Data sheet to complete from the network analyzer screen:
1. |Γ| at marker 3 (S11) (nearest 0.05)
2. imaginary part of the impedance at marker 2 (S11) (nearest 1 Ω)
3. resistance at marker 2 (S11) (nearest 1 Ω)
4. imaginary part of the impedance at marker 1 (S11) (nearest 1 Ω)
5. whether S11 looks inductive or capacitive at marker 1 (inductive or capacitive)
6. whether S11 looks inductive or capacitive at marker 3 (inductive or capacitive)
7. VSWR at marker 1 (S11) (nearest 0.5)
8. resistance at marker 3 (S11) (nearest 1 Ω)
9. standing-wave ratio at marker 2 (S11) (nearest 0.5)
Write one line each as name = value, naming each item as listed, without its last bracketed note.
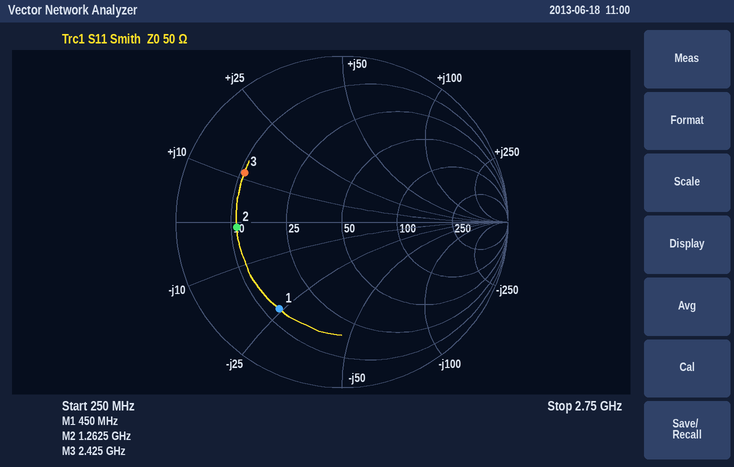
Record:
|Γ| at marker 3 (S11) = 0.65
imaginary part of the impedance at marker 2 (S11) = -1 Ω
resistance at marker 2 (S11) = 11 Ω
imaginary part of the impedance at marker 1 (S11) = -24 Ω
whether S11 looks inductive or capacitive at marker 1 = capacitive
whether S11 looks inductive or capacitive at marker 3 = inductive
VSWR at marker 1 (S11) = 4.5
resistance at marker 3 (S11) = 11 Ω
standing-wave ratio at marker 2 (S11) = 4.5
